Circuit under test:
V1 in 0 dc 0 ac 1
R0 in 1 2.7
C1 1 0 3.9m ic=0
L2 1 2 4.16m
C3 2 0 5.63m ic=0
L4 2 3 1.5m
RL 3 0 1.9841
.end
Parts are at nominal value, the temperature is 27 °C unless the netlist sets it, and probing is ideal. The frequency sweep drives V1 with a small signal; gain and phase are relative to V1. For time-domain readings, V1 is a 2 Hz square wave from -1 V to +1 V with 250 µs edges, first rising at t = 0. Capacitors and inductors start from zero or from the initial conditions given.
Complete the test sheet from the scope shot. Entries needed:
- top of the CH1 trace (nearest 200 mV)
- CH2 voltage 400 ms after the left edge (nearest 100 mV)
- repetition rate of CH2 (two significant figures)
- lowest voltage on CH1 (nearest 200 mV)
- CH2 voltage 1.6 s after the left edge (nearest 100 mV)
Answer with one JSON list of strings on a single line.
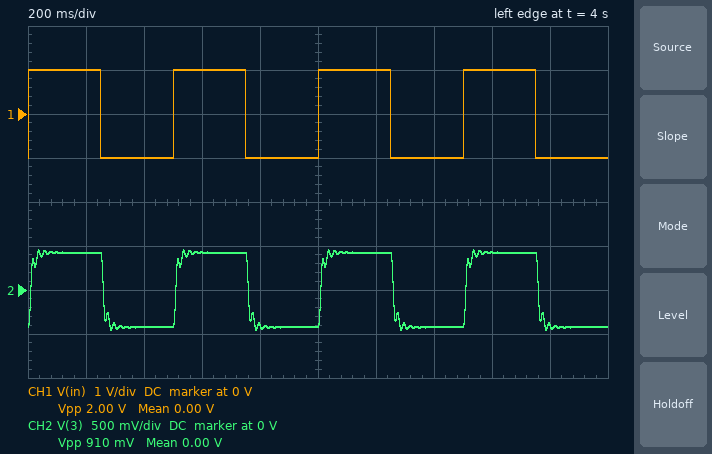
["1.0 V", "-400 mV", "2.0 Hz", "-1.0 V", "400 mV"]
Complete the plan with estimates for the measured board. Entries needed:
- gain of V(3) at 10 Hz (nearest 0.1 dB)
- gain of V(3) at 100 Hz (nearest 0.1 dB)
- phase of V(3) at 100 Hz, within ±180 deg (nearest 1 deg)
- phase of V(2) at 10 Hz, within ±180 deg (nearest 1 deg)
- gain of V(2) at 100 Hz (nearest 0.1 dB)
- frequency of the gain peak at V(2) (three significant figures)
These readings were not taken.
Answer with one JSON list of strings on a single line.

["-8.7 dB", "-33.6 dB", "83 deg", "-37 deg", "-32.7 dB", "50.0 Hz"]
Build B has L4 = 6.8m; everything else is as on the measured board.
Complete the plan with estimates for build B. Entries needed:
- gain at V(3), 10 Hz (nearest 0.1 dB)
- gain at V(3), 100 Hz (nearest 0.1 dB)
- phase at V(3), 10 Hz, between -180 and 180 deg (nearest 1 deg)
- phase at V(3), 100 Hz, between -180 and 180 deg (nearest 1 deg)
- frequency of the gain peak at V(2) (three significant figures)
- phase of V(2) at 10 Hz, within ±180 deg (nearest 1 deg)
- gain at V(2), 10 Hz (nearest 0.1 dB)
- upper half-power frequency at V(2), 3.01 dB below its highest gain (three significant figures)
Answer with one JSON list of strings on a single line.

["-8.4 dB", "-40.2 dB", "-46 deg", "37 deg", "51.8 Hz", "-33 deg", "-8.2 dB", "56.8 Hz"]
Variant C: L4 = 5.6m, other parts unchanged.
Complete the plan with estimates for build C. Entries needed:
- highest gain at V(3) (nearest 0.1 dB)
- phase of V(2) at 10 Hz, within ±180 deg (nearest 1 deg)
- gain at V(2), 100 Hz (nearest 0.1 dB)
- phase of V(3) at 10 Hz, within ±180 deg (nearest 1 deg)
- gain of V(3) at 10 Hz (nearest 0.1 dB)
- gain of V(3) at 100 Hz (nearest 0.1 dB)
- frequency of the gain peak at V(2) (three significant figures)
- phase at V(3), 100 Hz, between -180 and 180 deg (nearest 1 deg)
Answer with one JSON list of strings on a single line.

["-7.5 dB", "-34 deg", "-32.6 dB", "-44 deg", "-8.5 dB", "-38.8 dB", "51.7 Hz", "42 deg"]
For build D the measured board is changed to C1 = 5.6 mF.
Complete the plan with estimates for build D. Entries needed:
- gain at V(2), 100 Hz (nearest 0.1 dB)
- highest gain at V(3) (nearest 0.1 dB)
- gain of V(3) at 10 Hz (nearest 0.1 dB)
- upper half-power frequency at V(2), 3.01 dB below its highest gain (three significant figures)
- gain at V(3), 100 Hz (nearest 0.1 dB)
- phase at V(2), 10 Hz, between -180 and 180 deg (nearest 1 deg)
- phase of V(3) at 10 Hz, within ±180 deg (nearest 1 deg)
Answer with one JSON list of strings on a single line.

["-36.3 dB", "-7.5 dB", "-9.1 dB", "51.3 Hz", "-37.2 dB", "-41 deg", "-44 deg"]
